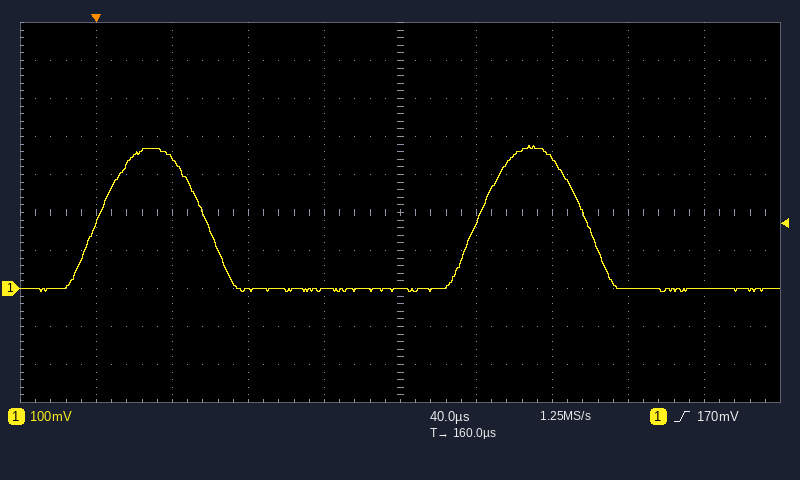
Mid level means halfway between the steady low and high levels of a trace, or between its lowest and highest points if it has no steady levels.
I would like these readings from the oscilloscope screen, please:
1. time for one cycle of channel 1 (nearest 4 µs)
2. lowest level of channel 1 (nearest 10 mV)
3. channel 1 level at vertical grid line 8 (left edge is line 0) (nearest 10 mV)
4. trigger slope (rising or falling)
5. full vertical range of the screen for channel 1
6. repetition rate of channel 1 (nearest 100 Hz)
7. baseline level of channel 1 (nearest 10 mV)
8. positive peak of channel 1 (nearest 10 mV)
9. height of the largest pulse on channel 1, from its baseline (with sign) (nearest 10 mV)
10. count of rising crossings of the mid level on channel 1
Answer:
200 µs
-10 mV
0 mV
rising
1 V
5.0 kHz
0 mV
380 mV
+380 mV
2
